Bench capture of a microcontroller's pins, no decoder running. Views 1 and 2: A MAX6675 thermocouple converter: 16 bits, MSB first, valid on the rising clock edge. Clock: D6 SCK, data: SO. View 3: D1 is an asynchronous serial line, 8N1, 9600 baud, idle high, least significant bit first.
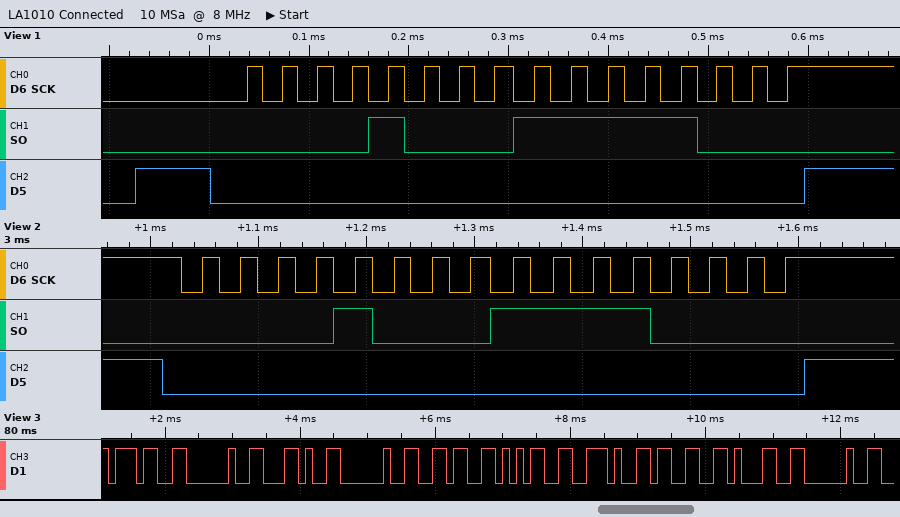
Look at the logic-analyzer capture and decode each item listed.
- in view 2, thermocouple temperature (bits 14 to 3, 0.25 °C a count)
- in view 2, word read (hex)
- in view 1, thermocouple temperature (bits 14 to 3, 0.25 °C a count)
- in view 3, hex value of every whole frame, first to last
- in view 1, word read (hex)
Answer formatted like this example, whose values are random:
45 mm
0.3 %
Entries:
71.50 °C
0x08F0
71.75 °C
37 20 2C 20 36 35 2E 33 31 20
0x08F8
